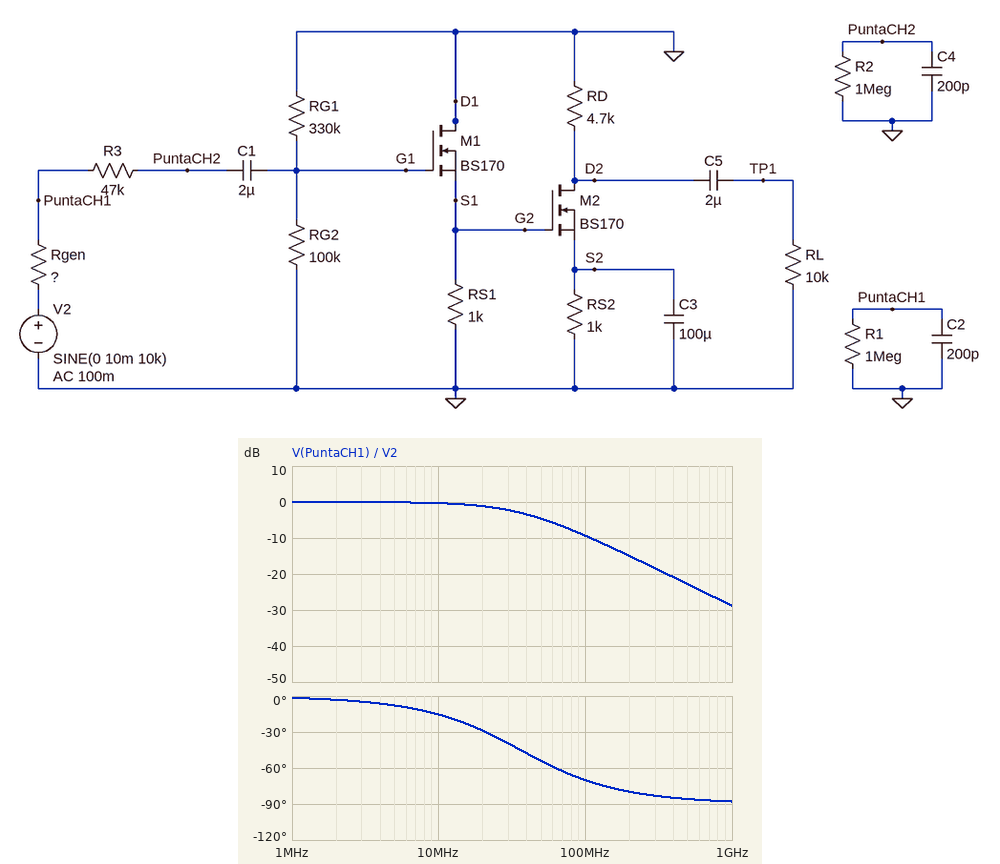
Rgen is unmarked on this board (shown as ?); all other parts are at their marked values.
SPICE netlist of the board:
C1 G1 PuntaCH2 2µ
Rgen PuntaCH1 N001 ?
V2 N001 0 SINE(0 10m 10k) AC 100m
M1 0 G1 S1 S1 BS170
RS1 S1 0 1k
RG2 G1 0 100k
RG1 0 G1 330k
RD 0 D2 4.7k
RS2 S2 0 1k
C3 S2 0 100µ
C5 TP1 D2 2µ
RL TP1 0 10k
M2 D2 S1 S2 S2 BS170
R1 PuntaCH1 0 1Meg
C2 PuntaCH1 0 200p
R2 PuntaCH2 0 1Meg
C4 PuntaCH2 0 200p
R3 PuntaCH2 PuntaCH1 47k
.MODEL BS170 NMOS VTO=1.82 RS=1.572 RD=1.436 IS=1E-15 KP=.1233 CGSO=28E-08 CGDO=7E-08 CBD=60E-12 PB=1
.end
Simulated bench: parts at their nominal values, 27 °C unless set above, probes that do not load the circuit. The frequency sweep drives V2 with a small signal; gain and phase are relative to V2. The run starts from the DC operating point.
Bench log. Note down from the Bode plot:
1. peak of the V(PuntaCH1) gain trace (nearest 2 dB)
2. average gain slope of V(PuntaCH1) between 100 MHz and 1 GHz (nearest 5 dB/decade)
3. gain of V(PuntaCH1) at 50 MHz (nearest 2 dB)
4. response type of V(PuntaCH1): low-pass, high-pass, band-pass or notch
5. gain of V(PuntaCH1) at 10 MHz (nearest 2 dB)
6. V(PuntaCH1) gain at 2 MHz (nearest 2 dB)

0 dB
-20 dB/decade
-4 dB
low-pass
0 dB
0 dB
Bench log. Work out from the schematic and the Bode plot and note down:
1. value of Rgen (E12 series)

22 Ω
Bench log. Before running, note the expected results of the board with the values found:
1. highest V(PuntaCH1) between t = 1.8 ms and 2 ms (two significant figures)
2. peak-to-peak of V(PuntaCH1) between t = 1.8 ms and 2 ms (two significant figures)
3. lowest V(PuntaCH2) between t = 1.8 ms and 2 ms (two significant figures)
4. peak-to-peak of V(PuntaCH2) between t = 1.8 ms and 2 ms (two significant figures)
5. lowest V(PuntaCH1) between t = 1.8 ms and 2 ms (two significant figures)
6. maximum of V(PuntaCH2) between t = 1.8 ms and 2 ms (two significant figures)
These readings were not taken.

10 mV
20 mV
-5.6 mV
11 mV
-10 mV
5.6 mV
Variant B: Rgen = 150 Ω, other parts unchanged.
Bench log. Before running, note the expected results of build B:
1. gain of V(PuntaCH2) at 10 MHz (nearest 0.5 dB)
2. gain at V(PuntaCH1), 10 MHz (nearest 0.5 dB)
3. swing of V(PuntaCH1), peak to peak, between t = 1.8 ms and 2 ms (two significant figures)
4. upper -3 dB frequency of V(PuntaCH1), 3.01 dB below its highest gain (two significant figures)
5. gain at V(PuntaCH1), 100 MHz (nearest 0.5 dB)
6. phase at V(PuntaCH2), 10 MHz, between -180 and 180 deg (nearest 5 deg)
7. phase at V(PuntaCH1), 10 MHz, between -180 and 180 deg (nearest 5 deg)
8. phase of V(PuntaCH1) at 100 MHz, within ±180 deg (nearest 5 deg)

-63.0 dB
-6.5 dB
20 mV
5.3 MHz
-25.5 dB
-150 deg
-60 deg
-85 deg
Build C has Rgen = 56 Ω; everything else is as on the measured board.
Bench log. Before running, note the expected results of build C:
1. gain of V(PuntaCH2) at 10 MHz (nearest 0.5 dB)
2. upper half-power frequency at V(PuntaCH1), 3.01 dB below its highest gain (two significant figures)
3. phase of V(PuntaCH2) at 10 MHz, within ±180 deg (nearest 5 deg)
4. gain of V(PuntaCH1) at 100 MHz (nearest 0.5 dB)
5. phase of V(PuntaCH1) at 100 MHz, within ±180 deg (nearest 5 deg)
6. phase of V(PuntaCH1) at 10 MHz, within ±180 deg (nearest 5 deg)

-58.5 dB
14 MHz
-125 deg
-17.0 dB
-80 deg
-35 deg
